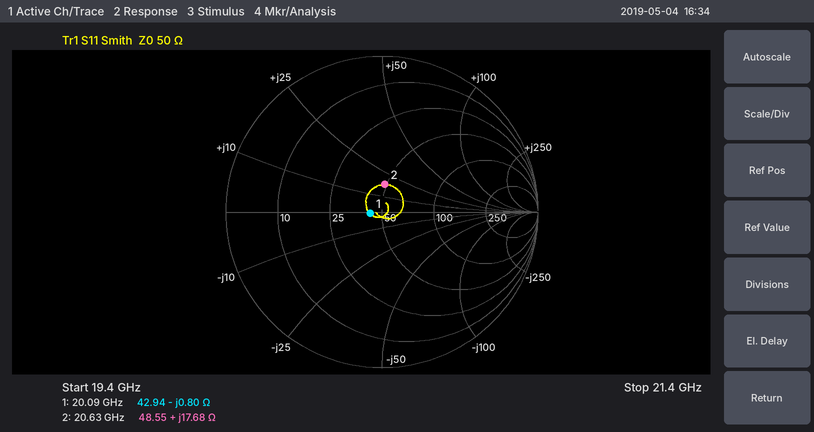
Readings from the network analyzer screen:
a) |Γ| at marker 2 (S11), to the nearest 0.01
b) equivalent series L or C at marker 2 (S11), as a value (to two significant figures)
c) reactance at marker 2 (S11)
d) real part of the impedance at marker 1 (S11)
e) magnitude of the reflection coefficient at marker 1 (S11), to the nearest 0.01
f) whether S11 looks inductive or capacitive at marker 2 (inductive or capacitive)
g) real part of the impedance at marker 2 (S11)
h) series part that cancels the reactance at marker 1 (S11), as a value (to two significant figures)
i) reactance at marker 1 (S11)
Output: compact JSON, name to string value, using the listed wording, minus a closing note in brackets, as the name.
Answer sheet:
{"|Γ| at marker 2 (S11), to the nearest 0.01": "0.18", "equivalent series L or C at marker 2 (S11), as a value": "140 pH", "reactance at marker 2": "+17.68 Ω", "real part of the impedance at marker 1": "42.94 Ω", "magnitude of the reflection coefficient at marker 1 (S11), to the nearest 0.01": "0.08", "whether S11 looks inductive or capacitive at marker 2": "inductive", "real part of the impedance at marker 2": "48.55 Ω", "series part that cancels the reactance at marker 1 (S11), as a value": "6.3 pH", "reactance at marker 1": "-0.80 Ω"}
